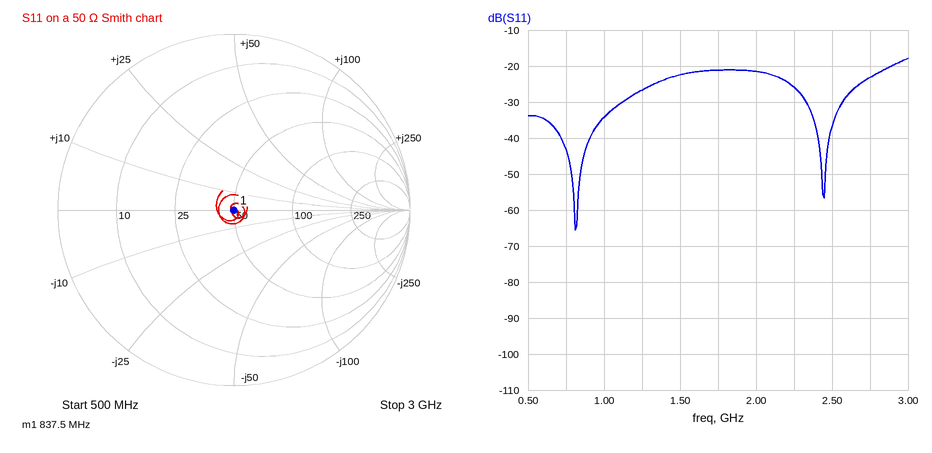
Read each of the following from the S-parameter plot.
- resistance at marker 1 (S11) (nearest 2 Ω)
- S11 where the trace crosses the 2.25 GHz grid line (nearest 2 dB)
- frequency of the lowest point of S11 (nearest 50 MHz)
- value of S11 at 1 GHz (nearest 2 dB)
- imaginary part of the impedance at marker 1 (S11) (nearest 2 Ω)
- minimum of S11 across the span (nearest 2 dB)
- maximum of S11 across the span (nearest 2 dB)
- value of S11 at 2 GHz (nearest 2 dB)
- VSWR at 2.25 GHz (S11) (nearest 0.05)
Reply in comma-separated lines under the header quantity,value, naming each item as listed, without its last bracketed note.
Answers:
quantity,value
resistance at marker 1 (S11),50 Ω
S11 where the trace crosses the 2.25 GHz grid line,-26 dB
frequency of the lowest point of S11,800 MHz
value of S11 at 1 GHz,-34 dB
imaginary part of the impedance at marker 1 (S11),0 Ω
minimum of S11 across the span,-66 dB
maximum of S11 across the span,-18 dB
value of S11 at 2 GHz,-22 dB
VSWR at 2.25 GHz (S11),1.10
